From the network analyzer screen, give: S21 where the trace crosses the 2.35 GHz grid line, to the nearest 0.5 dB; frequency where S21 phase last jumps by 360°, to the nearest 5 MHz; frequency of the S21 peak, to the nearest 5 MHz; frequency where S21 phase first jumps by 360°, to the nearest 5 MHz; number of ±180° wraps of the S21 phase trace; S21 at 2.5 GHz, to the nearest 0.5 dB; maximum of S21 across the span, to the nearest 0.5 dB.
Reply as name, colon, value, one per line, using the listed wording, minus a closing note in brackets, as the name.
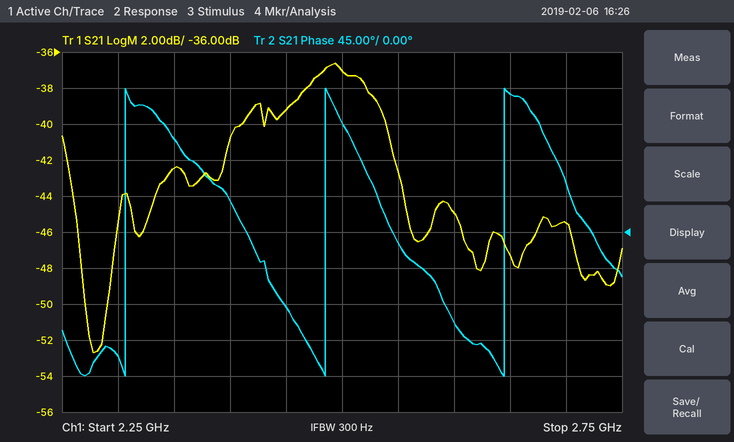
S21 where the trace crosses the 2.35 GHz grid line, to the nearest 0.5 dB: -42.5 dB
frequency where S21 phase last jumps by 360°, to the nearest 5 MHz: 2.645 GHz
frequency of the S21 peak, to the nearest 5 MHz: 2.495 GHz
frequency where S21 phase first jumps by 360°, to the nearest 5 MHz: 2.305 GHz
number of ±180° wraps of the S21 phase trace: 3
S21 at 2.5 GHz, to the nearest 0.5 dB: -37.0 dB
maximum of S21 across the span, to the nearest 0.5 dB: -36.5 dB
